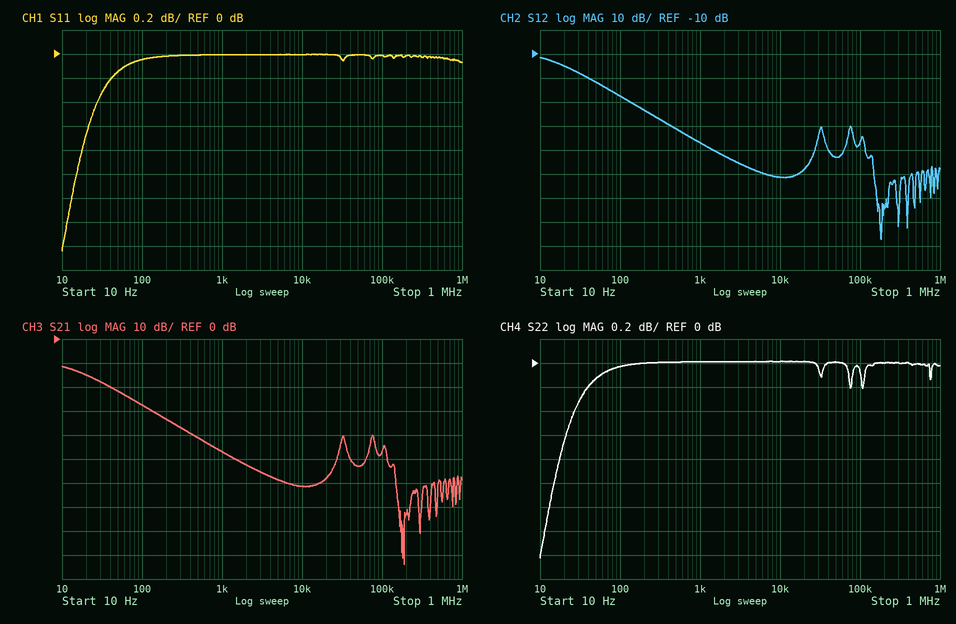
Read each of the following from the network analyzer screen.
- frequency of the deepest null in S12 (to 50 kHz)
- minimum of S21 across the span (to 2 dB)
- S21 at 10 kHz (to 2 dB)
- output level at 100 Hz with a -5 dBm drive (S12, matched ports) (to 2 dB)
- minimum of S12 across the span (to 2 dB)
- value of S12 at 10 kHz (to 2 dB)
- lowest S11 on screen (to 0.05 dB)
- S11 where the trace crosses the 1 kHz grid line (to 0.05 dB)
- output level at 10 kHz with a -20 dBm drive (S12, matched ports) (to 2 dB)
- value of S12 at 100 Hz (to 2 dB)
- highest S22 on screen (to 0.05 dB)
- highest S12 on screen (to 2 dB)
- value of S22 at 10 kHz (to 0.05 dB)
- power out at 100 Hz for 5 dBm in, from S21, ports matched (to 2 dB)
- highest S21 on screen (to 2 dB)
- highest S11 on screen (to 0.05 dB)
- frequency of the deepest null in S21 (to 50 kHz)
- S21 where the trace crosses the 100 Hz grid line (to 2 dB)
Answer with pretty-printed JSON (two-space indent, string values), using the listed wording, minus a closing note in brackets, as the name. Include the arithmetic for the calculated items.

{
  "frequency of the deepest null in S12": "200 kHz",
  "minimum of S21 across the span": "-94 dB",
  "S21 at 10 kHz": "-62 dB",
  "output level at 100 Hz with a -5 dBm drive (S12, matched ports)": "-5 dBm + (-28 dB) = -32 dBm",
  "minimum of S12 across the span": "-88 dB",
  "value of S12 at 10 kHz": "-62 dB",
  "lowest S11 on screen": "-1.65 dB",
  "S11 where the trace crosses the 1 kHz grid line": "0.00 dB",
  "output level at 10 kHz with a -20 dBm drive (S12, matched ports)": "-20 dBm + (-62 dB) = -82 dBm",
  "value of S12 at 100 Hz": "-28 dB",
  "highest S22 on screen": "0.00 dB",
  "highest S12 on screen": "-12 dB",
  "value of S22 at 10 kHz": "0.00 dB",
  "power out at 100 Hz for 5 dBm in, from S21, ports matched": "5 dBm + (-28 dB) = -22 dBm",
  "highest S21 on screen": "-12 dB",
  "highest S11 on screen": "0.00 dB",
  "frequency of the deepest null in S21": "200 kHz",
  "S21 where the trace crosses the 100 Hz grid line": "-28 dB"
}
